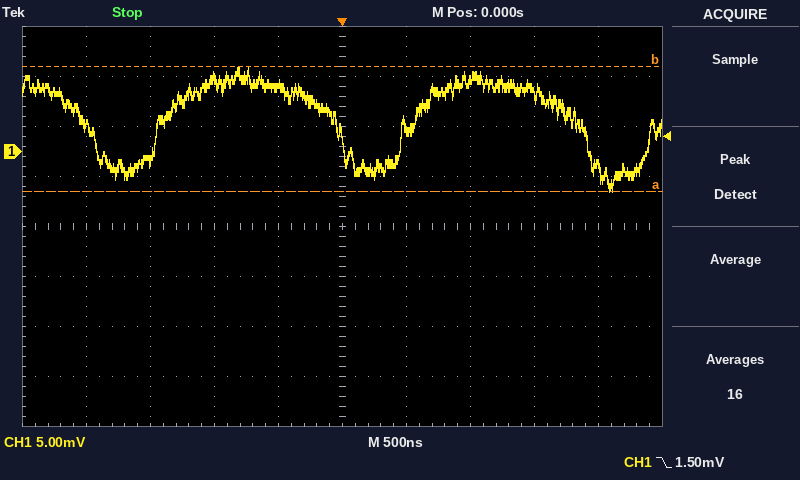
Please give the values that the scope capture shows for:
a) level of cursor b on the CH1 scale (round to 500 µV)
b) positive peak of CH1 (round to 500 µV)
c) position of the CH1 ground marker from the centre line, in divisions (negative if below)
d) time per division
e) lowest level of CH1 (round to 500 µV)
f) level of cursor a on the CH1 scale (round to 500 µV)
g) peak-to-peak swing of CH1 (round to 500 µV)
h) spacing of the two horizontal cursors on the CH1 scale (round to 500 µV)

8.5 mV
8.5 mV
+1.5 div
500 ns
-4.0 mV
-4.0 mV
12.5 mV
12.5 mV
